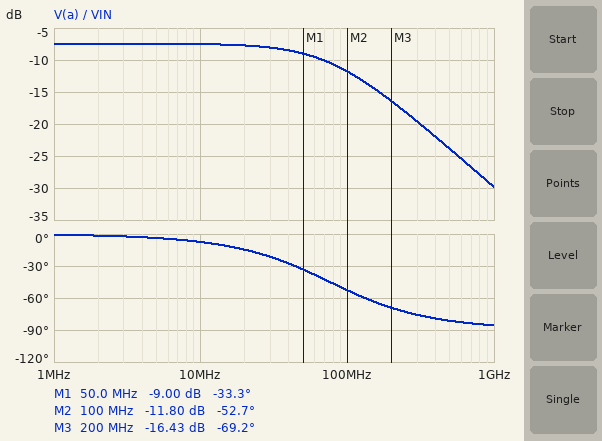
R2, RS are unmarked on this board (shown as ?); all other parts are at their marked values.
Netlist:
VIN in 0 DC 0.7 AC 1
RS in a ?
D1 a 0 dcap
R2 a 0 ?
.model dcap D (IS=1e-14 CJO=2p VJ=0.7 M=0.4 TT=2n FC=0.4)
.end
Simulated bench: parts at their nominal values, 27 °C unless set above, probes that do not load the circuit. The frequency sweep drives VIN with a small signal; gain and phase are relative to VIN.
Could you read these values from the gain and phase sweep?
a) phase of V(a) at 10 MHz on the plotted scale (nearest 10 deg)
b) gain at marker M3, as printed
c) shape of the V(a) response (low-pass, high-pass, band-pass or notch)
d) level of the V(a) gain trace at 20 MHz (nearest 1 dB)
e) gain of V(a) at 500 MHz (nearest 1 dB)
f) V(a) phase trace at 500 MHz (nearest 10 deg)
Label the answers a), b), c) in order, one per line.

a) -10 deg
b) -16.43 dB
c) low-pass
d) -8 dB
e) -24 dB
f) -80 deg
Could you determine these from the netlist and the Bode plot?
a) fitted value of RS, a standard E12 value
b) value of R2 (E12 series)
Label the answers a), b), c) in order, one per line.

a) 820 Ω
b) 4.7 kΩ
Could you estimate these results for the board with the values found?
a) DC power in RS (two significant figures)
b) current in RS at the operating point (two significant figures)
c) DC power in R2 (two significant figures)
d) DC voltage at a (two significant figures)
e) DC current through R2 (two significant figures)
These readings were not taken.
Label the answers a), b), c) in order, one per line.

a) 21 µW
b) 160 µA
c) 69 µW
d) 570 mV
e) 120 µA
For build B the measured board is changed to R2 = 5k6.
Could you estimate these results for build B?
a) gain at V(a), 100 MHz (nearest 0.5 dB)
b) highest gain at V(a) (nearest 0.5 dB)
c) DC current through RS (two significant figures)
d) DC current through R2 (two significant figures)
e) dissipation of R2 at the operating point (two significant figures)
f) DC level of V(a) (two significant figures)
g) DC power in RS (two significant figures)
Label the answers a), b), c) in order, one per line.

a) -13.0 dB
b) -8.5 dB
c) 150 µA
d) 100 µA
e) 59 µW
f) 580 mV
g) 19 µW
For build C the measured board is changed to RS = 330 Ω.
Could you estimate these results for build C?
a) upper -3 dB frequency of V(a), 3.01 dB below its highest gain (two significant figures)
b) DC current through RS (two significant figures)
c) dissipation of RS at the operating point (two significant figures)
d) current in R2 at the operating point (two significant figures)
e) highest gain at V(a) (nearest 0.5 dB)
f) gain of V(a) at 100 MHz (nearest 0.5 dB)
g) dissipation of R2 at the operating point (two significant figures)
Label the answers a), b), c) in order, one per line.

a) 97 MHz
b) 280 µA
c) 26 µW
d) 130 µA
e) -9.5 dB
f) -13.0 dB
g) 78 µW
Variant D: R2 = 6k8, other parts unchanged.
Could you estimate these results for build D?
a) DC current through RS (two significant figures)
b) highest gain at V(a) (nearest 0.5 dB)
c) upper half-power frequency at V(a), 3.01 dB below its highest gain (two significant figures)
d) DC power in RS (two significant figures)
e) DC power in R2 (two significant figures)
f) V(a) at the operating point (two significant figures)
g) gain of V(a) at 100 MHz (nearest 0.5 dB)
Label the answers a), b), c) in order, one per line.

a) 140 µA
b) -9.5 dB
c) 75 MHz
d) 17 µW
e) 50 µW
f) 580 mV
g) -14.0 dB
